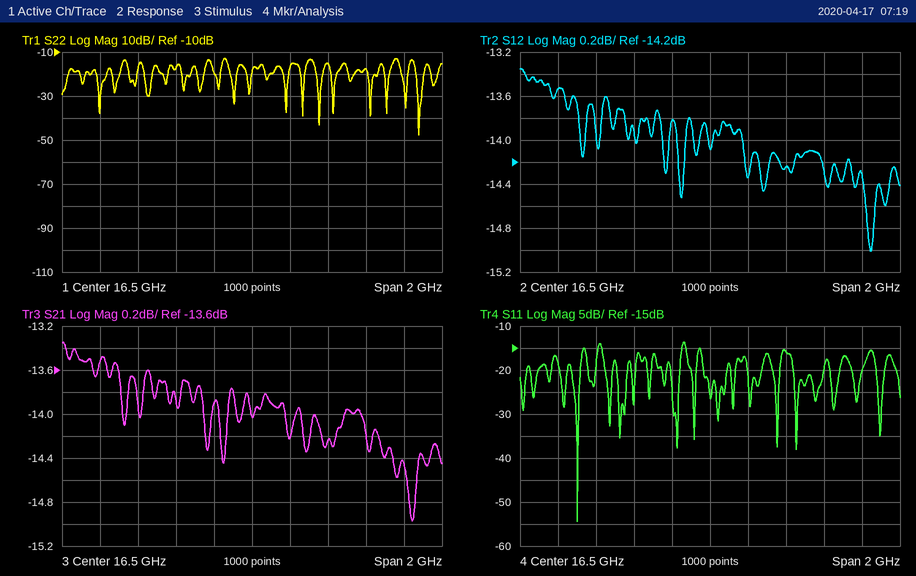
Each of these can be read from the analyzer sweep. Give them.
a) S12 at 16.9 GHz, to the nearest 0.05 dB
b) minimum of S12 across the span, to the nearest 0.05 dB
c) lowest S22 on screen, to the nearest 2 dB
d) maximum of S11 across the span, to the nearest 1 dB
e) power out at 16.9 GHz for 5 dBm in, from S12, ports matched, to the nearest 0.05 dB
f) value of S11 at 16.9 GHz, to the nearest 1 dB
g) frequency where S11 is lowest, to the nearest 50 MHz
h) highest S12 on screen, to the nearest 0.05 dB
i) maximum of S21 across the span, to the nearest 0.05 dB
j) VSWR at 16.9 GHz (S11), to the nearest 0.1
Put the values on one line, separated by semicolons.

-14.25 dB; -15.00 dB; -48 dB; -14 dB; -9.25 dBm; -16 dB; 15.80 GHz; -13.35 dB; -13.35 dB; 1.4
